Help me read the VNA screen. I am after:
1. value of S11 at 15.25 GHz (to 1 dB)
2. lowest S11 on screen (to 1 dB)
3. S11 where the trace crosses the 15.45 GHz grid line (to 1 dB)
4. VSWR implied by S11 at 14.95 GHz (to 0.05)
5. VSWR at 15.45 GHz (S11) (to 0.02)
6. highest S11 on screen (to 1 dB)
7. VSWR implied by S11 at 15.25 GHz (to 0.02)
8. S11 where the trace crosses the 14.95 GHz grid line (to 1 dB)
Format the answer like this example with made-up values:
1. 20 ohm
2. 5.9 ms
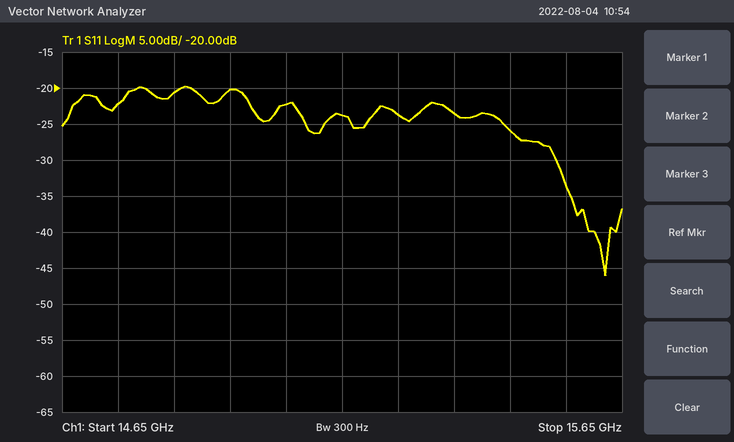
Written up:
1. -24 dB
2. -46 dB
3. -26 dB
4. 1.20
5. 1.10
6. -20 dB
7. 1.14
8. -20 dB
